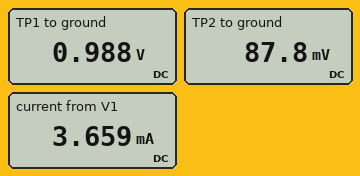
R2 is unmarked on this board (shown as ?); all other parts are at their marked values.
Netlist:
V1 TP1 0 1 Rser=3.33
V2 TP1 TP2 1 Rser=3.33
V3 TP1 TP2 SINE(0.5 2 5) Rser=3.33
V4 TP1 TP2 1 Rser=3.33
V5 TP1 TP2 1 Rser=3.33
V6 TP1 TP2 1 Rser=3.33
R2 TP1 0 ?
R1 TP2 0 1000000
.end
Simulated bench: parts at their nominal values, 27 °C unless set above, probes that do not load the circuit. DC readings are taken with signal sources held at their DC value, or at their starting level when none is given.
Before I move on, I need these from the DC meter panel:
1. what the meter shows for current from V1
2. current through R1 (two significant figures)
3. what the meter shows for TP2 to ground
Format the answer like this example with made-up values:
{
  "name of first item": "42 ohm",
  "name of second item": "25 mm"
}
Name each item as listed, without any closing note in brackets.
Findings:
{
  "what the meter shows for current from V1": "3.659 mA",
  "current through R1": "88 nA",
  "what the meter shows for TP2 to ground": "87.8 mV"
}
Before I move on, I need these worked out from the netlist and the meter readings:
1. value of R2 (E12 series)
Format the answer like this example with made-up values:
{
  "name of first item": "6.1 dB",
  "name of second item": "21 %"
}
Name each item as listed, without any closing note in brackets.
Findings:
{
  "value of R2": "270 Ω"
}
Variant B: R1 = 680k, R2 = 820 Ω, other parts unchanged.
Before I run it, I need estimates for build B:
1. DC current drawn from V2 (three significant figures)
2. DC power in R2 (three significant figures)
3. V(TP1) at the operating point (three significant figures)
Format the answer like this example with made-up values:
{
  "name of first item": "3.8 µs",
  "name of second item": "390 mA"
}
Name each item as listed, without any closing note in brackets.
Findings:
{
  "DC current drawn from V2": "30.0 mA",
  "DC power in R2": "1.21 mW",
  "V(TP1) at the operating point": "996 mV"
}
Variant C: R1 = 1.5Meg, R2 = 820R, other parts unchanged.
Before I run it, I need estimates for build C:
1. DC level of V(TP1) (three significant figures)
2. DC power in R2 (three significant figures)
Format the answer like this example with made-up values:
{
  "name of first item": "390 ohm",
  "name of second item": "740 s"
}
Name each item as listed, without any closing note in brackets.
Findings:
{
  "DC level of V(TP1)": "996 mV",
  "DC power in R2": "1.21 mW"
}
